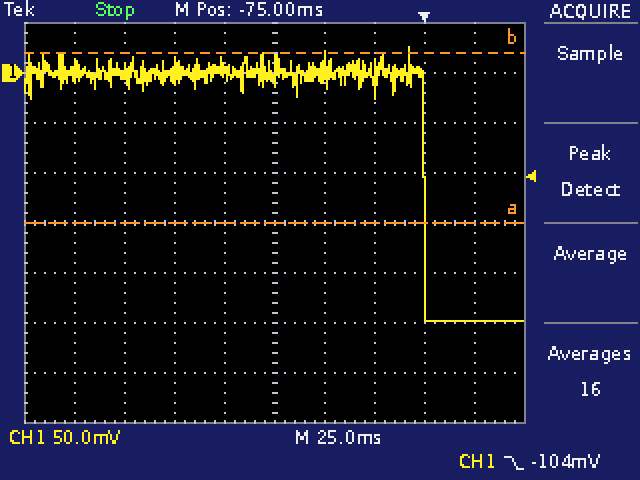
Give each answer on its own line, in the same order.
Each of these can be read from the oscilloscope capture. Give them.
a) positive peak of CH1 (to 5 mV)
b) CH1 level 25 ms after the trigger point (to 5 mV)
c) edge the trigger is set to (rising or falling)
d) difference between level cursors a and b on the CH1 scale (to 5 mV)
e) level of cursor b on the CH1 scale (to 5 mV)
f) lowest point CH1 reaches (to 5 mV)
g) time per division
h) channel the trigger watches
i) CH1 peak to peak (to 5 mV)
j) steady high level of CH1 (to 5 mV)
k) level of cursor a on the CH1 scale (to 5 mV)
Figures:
25 mV
-250 mV
falling
170 mV
20 mV
-250 mV
25 ms
CH1
275 mV
0 mV
-150 mV
